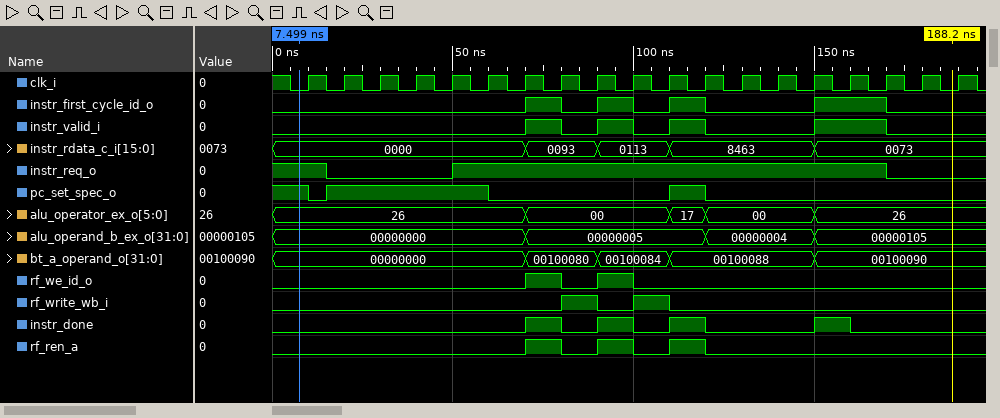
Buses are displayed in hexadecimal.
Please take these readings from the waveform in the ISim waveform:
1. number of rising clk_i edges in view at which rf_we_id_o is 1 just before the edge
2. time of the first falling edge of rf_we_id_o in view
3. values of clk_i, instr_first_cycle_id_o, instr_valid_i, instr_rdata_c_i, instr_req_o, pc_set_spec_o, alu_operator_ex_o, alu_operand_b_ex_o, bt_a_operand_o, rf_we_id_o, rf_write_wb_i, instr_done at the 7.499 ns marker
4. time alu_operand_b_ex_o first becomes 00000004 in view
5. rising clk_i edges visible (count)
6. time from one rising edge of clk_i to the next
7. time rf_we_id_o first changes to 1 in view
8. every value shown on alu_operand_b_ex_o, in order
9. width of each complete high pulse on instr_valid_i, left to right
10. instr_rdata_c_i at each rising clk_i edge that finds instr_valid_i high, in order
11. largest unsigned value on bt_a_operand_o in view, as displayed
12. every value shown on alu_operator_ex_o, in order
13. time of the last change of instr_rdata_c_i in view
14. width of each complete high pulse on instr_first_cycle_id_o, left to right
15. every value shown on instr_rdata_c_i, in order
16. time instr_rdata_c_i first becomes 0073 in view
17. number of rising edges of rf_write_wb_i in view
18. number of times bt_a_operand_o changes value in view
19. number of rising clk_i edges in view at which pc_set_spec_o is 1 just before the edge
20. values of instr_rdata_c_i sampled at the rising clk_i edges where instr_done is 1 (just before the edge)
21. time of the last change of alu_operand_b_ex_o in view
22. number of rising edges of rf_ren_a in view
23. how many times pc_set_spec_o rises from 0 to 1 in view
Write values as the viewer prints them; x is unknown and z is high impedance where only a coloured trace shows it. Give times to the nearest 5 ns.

2
80 ns
clk_i=0, instr_first_cycle_id_o=0, instr_valid_i=0, instr_rdata_c_i=0000, instr_req_o=1, pc_set_spec_o=1, alu_operator_ex_o=26, alu_operand_b_ex_o=00000000, bt_a_operand_o=00000000, rf_we_id_o=0, rf_write_wb_i=0, instr_done=0
120 ns
19
10 ns
70 ns
00000000, 00000005, 00000004, 00000105
10 ns, 10 ns, 10 ns, 20 ns
0093, 0113, 8463, 0073, 0073
00100090
26, 00, 17, 00, 26
150 ns
10 ns, 10 ns, 10 ns, 20 ns
0000, 0093, 0113, 8463, 0073
150 ns
2
4
7
0093, 0113, 8463, 0073
150 ns
3
2
